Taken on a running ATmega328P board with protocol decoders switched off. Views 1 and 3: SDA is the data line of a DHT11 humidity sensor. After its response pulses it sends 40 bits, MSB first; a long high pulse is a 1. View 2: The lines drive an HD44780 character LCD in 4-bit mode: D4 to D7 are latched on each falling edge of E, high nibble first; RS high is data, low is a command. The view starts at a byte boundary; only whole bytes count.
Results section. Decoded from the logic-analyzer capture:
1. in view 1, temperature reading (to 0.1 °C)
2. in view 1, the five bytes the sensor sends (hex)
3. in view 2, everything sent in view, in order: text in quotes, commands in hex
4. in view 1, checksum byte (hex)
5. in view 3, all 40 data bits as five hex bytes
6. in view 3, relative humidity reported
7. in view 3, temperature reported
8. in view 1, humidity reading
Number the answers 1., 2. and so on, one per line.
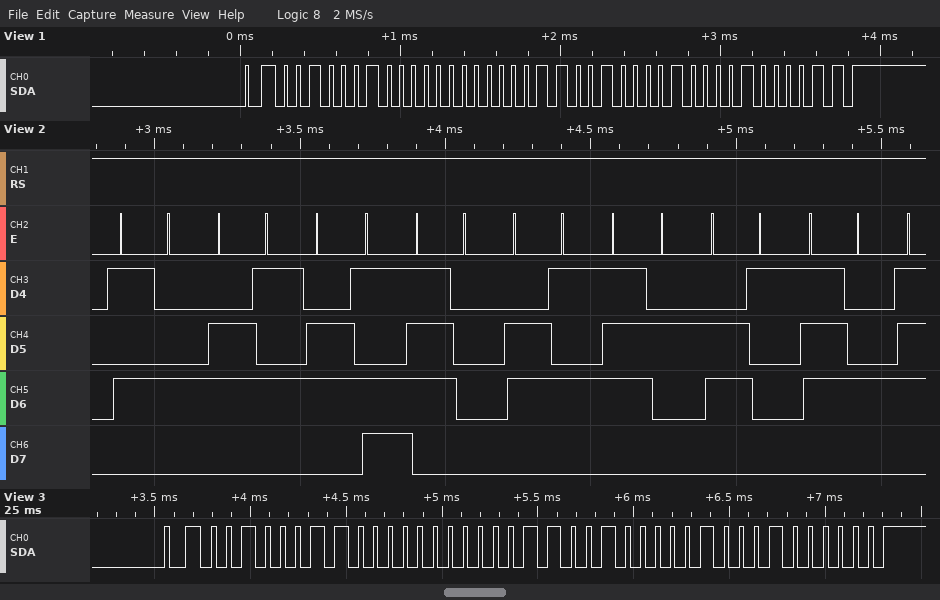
1. 25.8 °C
2. 22 00 19 08 43
3. "Temperat"
4. 0x43
5. 23 00 19 04 40
6. 35 %
7. 25.4 °C
8. 34 %
